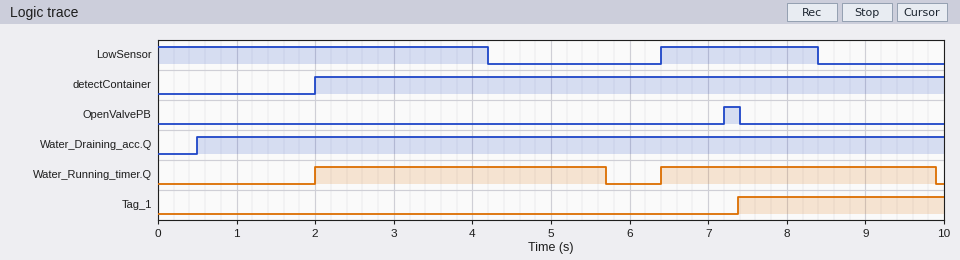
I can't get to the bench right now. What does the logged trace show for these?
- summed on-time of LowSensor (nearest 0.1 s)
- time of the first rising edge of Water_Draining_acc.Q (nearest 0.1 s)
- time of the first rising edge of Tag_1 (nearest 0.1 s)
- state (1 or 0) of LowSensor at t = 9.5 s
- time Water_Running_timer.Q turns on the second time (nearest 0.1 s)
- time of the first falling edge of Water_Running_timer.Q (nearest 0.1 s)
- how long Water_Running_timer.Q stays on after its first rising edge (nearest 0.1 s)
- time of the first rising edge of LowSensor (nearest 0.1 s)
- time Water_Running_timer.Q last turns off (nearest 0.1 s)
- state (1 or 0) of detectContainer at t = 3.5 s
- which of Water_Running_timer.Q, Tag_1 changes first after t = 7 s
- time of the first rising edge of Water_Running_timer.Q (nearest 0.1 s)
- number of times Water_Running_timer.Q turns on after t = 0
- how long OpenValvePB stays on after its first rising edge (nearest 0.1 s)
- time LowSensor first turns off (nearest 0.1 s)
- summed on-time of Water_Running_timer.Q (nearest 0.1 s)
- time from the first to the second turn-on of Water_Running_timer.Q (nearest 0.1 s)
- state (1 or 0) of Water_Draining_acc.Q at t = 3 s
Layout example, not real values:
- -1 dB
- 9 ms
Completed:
- 6.2 s
- 0.5 s
- 7.4 s
- 0
- 6.4 s
- 5.7 s
- 3.7 s
- 6.4 s
- 9.9 s
- 1
- Tag_1
- 2.0 s
- 2
- 0.2 s
- 4.2 s
- 7.2 s
- 4.4 s
- 1
